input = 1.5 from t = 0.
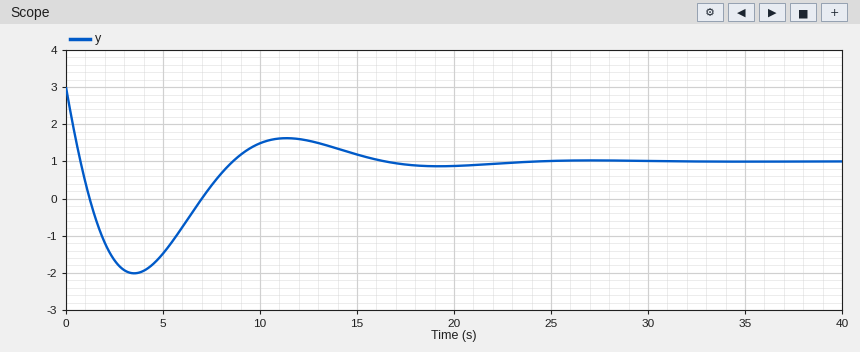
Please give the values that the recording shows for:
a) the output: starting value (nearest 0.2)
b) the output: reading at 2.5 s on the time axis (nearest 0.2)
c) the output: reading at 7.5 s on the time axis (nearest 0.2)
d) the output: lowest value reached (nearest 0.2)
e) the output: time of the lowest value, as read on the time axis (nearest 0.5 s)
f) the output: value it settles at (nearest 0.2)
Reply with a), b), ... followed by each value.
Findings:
a) 3.0
b) -1.6
c) 0.4
d) -2.0
e) 3.5 s
f) 1.0
